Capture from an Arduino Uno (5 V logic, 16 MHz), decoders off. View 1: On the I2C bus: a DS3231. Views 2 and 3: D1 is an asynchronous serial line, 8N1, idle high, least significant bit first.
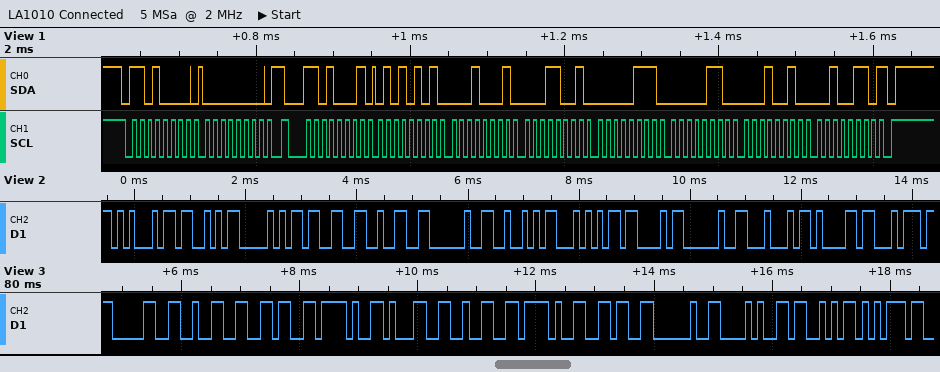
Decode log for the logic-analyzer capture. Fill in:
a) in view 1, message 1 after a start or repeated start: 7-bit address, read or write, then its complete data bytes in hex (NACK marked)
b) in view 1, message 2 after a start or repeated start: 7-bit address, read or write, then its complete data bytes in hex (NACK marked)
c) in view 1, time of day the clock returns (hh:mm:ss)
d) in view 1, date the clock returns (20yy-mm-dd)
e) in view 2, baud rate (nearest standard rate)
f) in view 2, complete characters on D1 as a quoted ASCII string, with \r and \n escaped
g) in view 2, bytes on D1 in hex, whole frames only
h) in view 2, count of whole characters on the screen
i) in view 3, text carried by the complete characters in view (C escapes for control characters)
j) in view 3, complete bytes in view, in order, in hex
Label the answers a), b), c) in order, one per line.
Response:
a) 0x68 write: 00
b) 0x68 read: 55 11 19 07 06 12 26 NACK
c) 19:11:55
d) 2026-12-06
e) 9600 baud
f) "ESP32 RTC Dat"
g) 45 53 50 33 32 20 52 54 43 20 44 61 74
h) 13
i) "026/12/6 (Su"
j) 30 32 36 2F 31 32 2F 36 20 28 53 75
